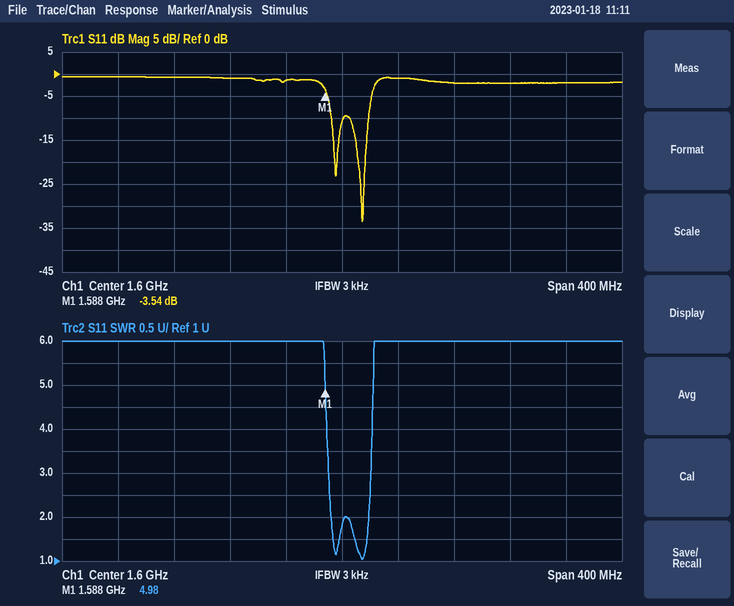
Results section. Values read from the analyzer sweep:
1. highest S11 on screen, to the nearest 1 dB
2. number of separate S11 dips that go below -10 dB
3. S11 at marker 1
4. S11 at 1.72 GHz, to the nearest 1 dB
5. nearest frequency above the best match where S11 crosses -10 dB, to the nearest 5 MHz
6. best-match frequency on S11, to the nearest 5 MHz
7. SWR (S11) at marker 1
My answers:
-1 dB
2
-3.54 dB
-2 dB
1.620 GHz
1.615 GHz
4.98
